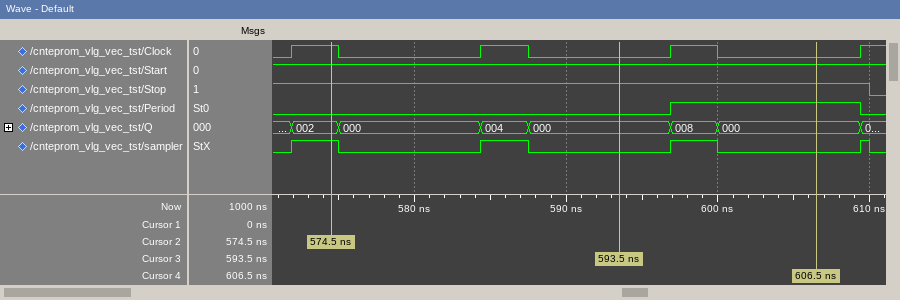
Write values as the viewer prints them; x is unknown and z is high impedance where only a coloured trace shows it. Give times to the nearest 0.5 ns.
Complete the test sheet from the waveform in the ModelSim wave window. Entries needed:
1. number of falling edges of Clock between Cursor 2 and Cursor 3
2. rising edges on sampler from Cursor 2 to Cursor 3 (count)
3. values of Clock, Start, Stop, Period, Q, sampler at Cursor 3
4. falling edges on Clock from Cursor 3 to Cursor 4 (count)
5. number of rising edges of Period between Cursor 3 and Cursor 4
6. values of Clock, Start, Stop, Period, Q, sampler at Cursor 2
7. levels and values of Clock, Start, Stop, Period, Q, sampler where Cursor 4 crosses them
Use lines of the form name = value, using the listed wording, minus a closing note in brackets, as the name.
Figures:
number of falling edges of Clock between Cursor 2 and Cursor 3 = 2
rising edges on sampler from Cursor 2 to Cursor 3 = 1
values of Clock, Start, Stop, Period, Q, sampler at Cursor 3 = Clock=0, Start=1, Stop=1, Period=0, Q=000, sampler=0
falling edges on Clock from Cursor 3 to Cursor 4 = 1
number of rising edges of Period between Cursor 3 and Cursor 4 = 1
values of Clock, Start, Stop, Period, Q, sampler at Cursor 2 = Clock=1, Start=1, Stop=1, Period=0, Q=002, sampler=1
levels and values of Clock, Start, Stop, Period, Q, sampler where Cursor 4 crosses them = Clock=0, Start=1, Stop=1, Period=1, Q=000, sampler=0
